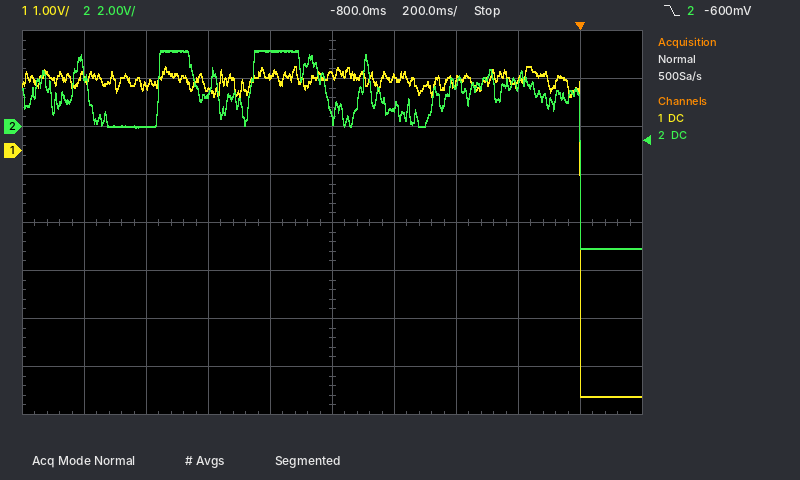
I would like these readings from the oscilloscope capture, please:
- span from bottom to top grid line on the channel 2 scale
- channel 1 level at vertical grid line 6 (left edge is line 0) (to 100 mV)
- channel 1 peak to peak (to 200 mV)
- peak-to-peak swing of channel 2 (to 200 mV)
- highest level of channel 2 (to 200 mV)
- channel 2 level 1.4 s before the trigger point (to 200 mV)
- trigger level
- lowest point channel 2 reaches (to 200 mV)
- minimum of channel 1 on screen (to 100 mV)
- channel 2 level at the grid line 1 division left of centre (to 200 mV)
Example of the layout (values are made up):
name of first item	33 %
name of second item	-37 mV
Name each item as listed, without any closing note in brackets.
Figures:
span from bottom to top grid line on the channel 2 scale	16 V
channel 1 level at vertical grid line 6 (left edge is line 0)	1.5 V
channel 1 peak to peak	6.8 V
peak-to-peak swing of channel 2	8.2 V
highest level of channel 2	3.2 V
channel 2 level 1.4 s before the trigger point	0.0 V
trigger level	-600 mV
lowest point channel 2 reaches	-5.0 V
minimum of channel 1 on screen	-5.1 V
channel 2 level at the grid line 1 division left of centre	3.2 V
